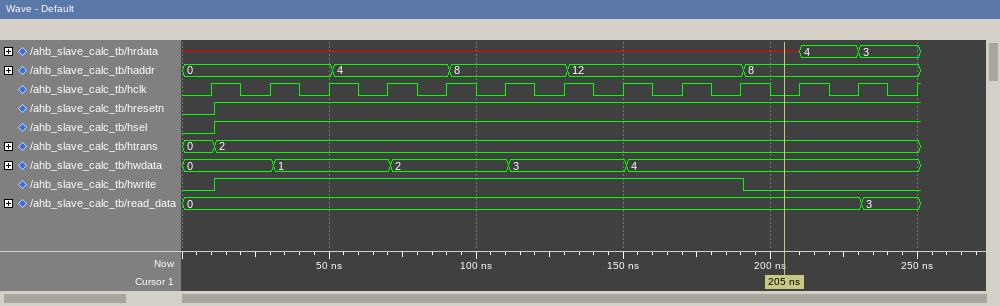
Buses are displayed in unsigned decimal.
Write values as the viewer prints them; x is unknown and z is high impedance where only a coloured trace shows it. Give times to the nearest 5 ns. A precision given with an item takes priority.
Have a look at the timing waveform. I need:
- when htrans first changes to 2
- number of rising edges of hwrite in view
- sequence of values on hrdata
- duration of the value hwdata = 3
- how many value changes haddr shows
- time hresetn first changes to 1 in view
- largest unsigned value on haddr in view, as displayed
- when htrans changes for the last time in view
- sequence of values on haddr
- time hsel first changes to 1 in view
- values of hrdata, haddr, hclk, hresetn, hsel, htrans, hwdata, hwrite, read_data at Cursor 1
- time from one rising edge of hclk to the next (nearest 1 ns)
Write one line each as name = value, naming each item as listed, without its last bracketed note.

when htrans first changes to 2 = 10 ns
number of rising edges of hwrite in view = 1
sequence of values on hrdata = x, 4, 3
duration of the value hwdata = 3 = 40 ns
how many value changes haddr shows = 4
time hresetn first changes to 1 in view = 10 ns
largest unsigned value on haddr in view, as displayed = 12
when htrans changes for the last time in view = 10 ns
sequence of values on haddr = 0, 4, 8, 12, 8
time hsel first changes to 1 in view = 10 ns
values of hrdata, haddr, hclk, hresetn, hsel, htrans, hwdata, hwrite, read_data at Cursor 1 = hrdata=x, haddr=8, hclk=0, hresetn=1, hsel=1, htrans=2, hwdata=4, hwrite=0, read_data=0
time from one rising edge of hclk to the next = 20 ns
